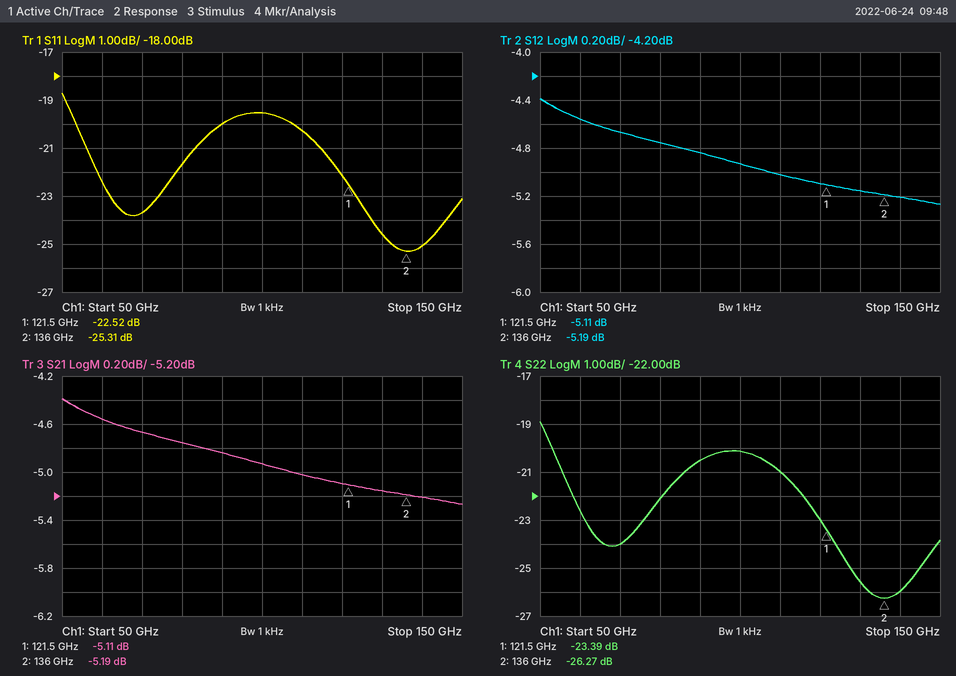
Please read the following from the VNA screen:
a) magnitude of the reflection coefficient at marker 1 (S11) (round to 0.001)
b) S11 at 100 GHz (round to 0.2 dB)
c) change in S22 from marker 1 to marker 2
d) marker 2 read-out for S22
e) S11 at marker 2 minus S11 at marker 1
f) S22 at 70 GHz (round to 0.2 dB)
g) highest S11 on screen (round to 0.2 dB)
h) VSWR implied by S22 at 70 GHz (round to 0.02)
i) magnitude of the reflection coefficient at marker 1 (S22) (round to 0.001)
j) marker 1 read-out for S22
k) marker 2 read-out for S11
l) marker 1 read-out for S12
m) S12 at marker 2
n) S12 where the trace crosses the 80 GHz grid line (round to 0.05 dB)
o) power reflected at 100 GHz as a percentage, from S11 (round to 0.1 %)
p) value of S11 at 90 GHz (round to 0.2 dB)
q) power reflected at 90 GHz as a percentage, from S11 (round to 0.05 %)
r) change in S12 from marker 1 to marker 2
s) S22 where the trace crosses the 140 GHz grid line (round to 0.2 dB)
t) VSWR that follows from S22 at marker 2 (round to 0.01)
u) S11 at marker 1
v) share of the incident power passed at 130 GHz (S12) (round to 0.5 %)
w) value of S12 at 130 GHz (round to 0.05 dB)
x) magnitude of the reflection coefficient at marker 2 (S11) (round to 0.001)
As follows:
0.075
-19.6 dB
-2.88 dB
-26.27 dB
-2.79 dB
-24.0 dB
-18.8 dB
1.14
0.068
-23.39 dB
-25.31 dB
-5.11 dB
-5.19 dB
-4.75 dB
1.1 %
-20.0 dB
1.00 %
-0.08 dB
-26.0 dB
1.10
-22.52 dB
30.5 %
-5.15 dB
0.054
